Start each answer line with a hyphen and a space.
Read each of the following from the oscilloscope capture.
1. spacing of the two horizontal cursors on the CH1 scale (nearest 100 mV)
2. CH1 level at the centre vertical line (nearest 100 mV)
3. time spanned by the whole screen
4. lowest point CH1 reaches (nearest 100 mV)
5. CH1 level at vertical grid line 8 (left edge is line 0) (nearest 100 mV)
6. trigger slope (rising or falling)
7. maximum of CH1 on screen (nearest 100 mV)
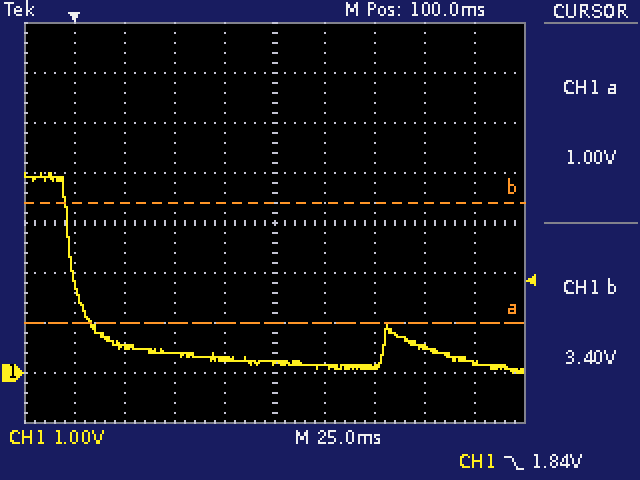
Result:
- 2.4 V
- 200 mV
- 250 ms
- 0.0 V
- 500 mV
- falling
- 4.0 V
